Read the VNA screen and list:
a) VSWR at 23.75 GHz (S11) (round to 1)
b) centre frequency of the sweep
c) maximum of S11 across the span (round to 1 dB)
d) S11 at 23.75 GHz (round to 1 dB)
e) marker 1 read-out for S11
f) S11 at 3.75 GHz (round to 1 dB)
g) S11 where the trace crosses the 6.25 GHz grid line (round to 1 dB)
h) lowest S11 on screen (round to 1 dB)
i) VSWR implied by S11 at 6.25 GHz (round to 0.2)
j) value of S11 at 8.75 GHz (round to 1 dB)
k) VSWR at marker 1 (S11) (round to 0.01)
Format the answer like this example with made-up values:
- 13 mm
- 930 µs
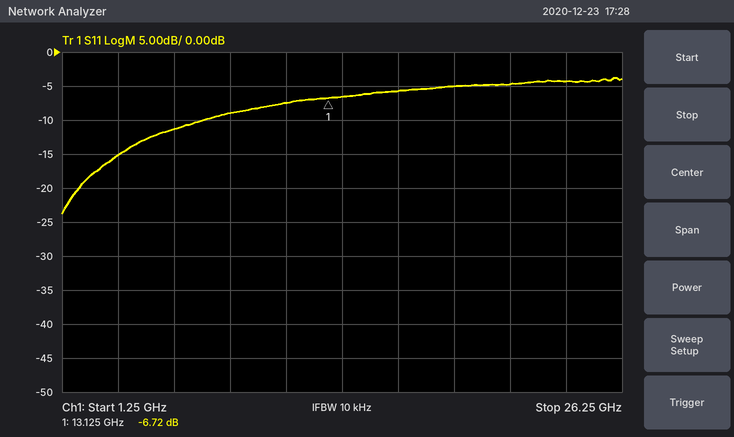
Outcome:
- 4
- 13.75 GHz
- -4 dB
- -4 dB
- -6.72 dB
- -15 dB
- -11 dB
- -24 dB
- 1.8
- -9 dB
- 2.71
